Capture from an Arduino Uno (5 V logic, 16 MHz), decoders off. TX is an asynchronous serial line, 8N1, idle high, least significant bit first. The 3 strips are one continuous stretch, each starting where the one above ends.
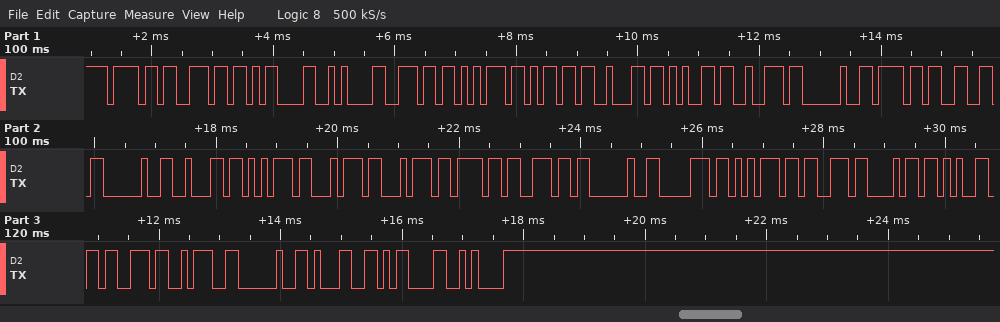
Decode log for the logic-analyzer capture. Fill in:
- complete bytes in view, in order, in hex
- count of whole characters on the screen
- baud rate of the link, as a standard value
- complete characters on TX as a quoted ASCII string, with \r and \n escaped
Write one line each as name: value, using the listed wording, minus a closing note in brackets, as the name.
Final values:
complete bytes in view, in order, in hex: 6F 6E 0D 0A 6E 75 6D 62 65 72 20 6F 66 20 62 75 74 74 6F 6E 20 70 75 73 68 65 73 3A 20 31 0D 0A
count of whole characters on the screen: 32
baud rate of the link, as a standard value: 9600 baud
complete characters on TX as a quoted ASCII string, with \r and \n escaped: "on\r\nnumber of button pushes: 1\r\n"
